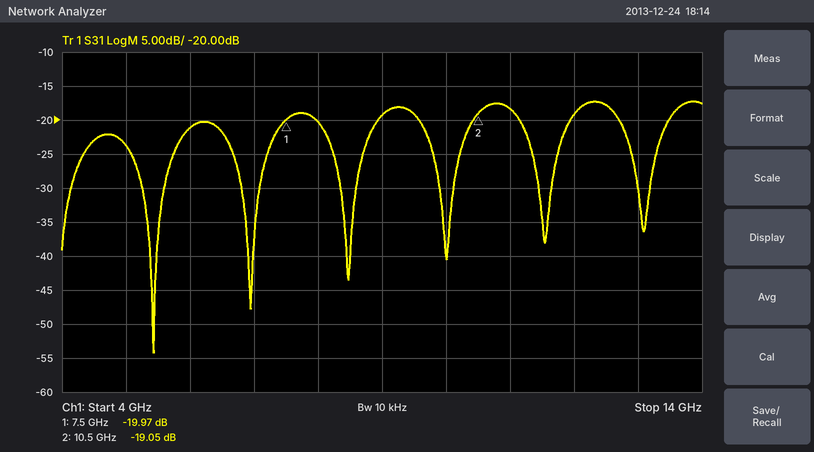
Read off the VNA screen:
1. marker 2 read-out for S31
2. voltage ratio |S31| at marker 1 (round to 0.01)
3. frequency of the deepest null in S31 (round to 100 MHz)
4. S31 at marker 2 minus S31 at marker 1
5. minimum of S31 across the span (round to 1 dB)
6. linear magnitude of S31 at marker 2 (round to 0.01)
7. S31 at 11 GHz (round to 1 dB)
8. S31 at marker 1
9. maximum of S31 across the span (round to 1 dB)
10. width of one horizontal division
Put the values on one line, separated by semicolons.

-19.05 dB; 0.10; 5.4 GHz; 0.92 dB; -54 dB; 0.11; -18 dB; -19.97 dB; -17 dB; 1 GHz
